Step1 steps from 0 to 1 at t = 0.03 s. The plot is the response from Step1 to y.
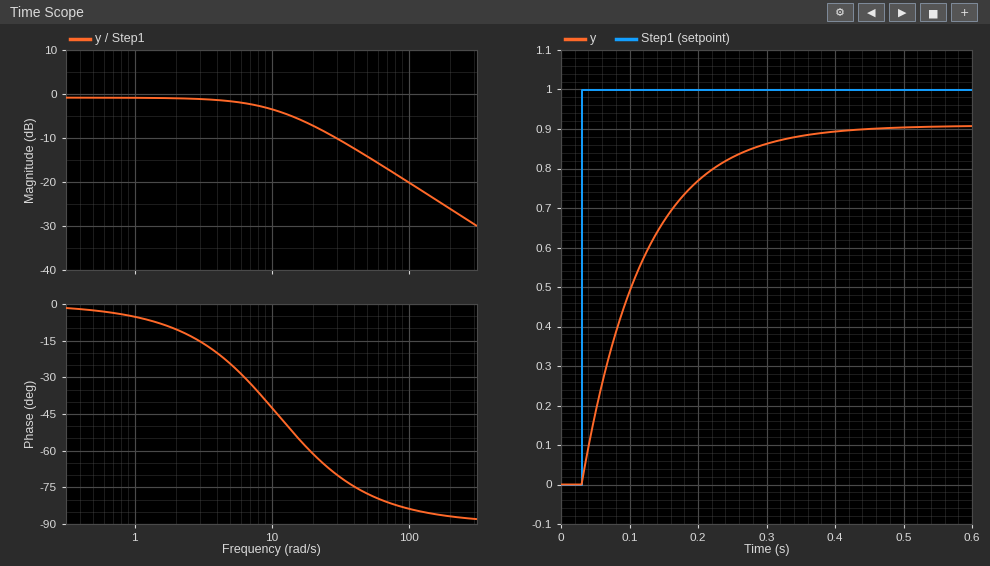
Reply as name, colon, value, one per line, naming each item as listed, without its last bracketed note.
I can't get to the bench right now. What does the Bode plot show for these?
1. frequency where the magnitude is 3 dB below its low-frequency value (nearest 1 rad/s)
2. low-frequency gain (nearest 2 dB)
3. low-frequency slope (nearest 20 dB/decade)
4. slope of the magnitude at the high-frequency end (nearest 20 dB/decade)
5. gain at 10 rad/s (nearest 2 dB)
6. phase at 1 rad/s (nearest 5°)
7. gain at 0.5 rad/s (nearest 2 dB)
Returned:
frequency where the magnitude is 3 dB below its low-frequency value: 11 rad/s
low-frequency gain: 0 dB
low-frequency slope: 0 dB/decade
slope of the magnitude at the high-frequency end: -20 dB/decade
gain at 10 rad/s: -4 dB
phase at 1 rad/s: -5°
gain at 0.5 rad/s: 0 dB
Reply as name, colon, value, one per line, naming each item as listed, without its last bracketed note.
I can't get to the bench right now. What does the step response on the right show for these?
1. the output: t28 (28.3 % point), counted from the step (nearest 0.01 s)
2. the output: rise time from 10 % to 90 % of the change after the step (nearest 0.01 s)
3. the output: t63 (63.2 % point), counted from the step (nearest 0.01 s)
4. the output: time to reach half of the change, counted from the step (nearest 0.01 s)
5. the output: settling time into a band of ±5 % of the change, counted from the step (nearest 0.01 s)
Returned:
the output: t28 (28.3 % point), counted from the step: 0.03 s
the output: rise time from 10 % to 90 % of the change after the step: 0.20 s
the output: t63 (63.2 % point), counted from the step: 0.09 s
the output: time to reach half of the change, counted from the step: 0.06 s
the output: settling time into a band of ±5 % of the change, counted from the step: 0.27 s
